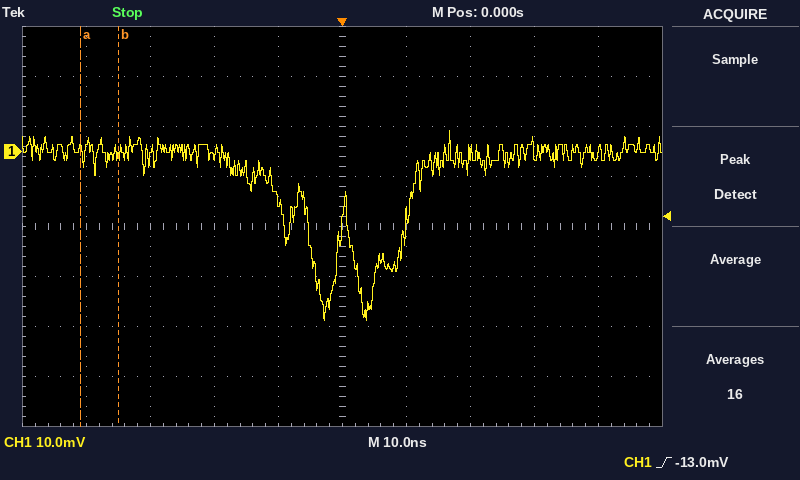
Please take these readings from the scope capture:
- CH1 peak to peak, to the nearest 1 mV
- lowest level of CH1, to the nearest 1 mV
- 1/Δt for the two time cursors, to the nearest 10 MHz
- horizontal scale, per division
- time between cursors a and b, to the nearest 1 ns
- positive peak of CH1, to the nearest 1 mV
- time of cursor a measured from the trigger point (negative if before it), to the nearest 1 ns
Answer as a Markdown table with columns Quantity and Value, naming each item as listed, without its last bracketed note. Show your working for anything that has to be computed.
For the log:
| Quantity | Value |
|---|---|
| CH1 peak to peak, to the nearest 1 mV | 4 mV − (-34 mV) = 38 mV |
| lowest level of CH1, to the nearest 1 mV | -34 mV |
| 1/Δt for the two time cursors, to the nearest 10 MHz | 1 / 6 ns ≈ 170 MHz |
| horizontal scale, per division | 10 ns |
| time between cursors a and b, to the nearest 1 ns | 6 ns |
| positive peak of CH1, to the nearest 1 mV | 4 mV |
| time of cursor a measured from the trigger point (negative if before it), to the nearest 1 ns | -41 ns |
